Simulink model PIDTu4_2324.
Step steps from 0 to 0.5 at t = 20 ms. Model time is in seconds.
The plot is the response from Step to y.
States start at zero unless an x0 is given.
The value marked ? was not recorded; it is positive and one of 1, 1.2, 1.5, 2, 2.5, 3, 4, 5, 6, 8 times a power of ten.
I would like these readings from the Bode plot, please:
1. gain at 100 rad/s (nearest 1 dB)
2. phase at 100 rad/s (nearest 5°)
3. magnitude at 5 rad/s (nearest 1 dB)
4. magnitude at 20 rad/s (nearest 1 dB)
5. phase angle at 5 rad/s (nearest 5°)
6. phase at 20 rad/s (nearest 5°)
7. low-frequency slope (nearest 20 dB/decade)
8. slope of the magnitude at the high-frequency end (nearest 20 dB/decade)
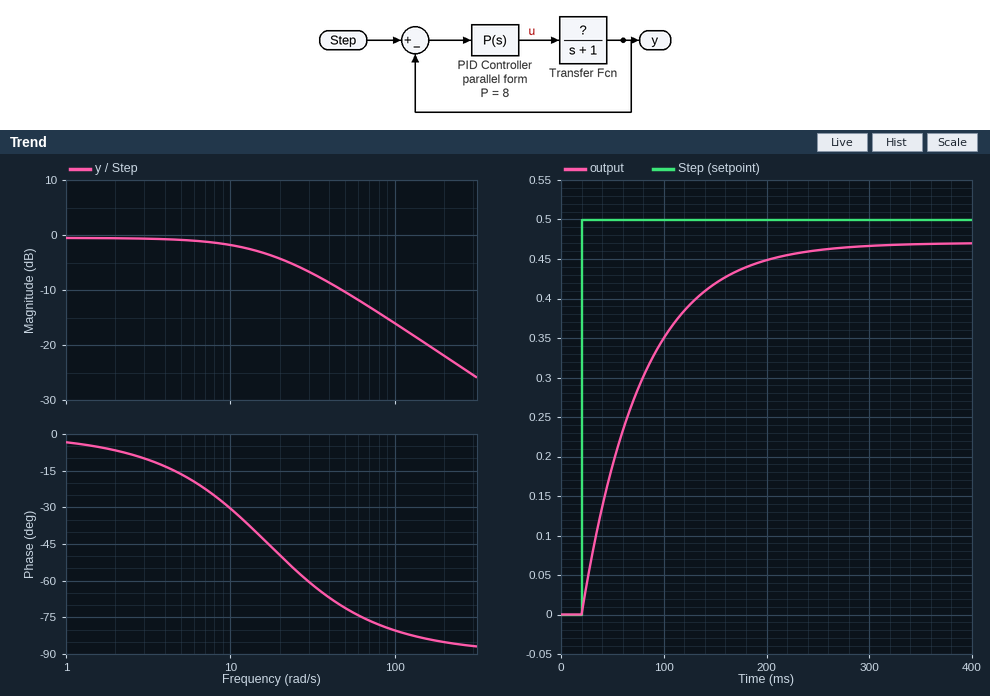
-16 dB
-80°
-1 dB
-4 dB
-15°
-50°
0 dB/decade
-20 dB/decade
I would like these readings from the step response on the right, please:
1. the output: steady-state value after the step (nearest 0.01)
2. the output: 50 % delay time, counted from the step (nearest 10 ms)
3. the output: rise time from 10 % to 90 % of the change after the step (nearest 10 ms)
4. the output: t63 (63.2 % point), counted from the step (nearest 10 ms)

0.47
40 ms
130 ms
60 ms
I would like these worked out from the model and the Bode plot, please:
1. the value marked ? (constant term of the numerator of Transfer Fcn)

2
